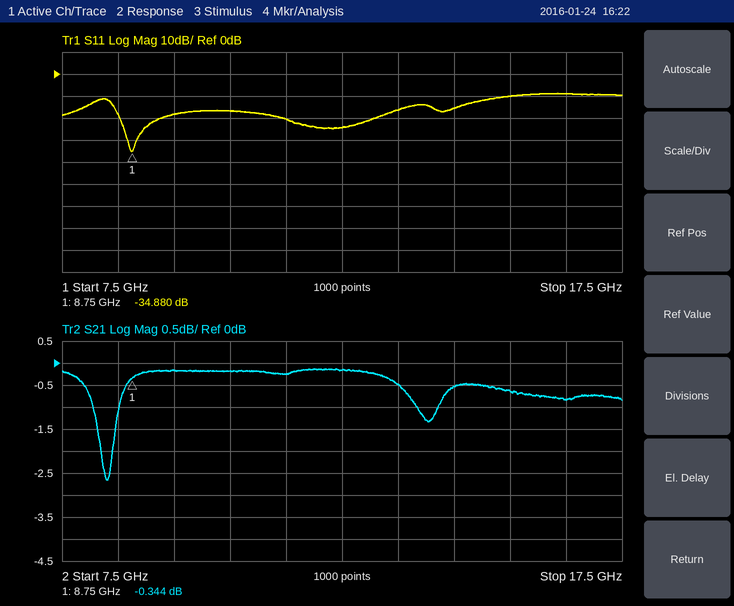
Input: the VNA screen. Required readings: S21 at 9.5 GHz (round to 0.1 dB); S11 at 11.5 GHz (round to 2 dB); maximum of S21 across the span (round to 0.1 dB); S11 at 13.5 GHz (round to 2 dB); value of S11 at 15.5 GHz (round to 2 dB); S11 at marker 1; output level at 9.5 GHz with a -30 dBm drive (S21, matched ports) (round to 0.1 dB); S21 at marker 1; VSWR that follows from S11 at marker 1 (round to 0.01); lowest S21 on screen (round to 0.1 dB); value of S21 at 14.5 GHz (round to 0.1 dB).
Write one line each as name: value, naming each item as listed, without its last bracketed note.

S21 at 9.5 GHz: -0.2 dB
S11 at 11.5 GHz: -20 dB
maximum of S21 across the span: -0.1 dB
S11 at 13.5 GHz: -16 dB
value of S11 at 15.5 GHz: -10 dB
S11 at marker 1: -34.880 dB
output level at 9.5 GHz with a -30 dBm drive (S21, matched ports): -30.2 dBm
S21 at marker 1: -0.344 dB
VSWR that follows from S11 at marker 1: 1.04
lowest S21 on screen: -2.7 dB
value of S21 at 14.5 GHz: -0.5 dB
